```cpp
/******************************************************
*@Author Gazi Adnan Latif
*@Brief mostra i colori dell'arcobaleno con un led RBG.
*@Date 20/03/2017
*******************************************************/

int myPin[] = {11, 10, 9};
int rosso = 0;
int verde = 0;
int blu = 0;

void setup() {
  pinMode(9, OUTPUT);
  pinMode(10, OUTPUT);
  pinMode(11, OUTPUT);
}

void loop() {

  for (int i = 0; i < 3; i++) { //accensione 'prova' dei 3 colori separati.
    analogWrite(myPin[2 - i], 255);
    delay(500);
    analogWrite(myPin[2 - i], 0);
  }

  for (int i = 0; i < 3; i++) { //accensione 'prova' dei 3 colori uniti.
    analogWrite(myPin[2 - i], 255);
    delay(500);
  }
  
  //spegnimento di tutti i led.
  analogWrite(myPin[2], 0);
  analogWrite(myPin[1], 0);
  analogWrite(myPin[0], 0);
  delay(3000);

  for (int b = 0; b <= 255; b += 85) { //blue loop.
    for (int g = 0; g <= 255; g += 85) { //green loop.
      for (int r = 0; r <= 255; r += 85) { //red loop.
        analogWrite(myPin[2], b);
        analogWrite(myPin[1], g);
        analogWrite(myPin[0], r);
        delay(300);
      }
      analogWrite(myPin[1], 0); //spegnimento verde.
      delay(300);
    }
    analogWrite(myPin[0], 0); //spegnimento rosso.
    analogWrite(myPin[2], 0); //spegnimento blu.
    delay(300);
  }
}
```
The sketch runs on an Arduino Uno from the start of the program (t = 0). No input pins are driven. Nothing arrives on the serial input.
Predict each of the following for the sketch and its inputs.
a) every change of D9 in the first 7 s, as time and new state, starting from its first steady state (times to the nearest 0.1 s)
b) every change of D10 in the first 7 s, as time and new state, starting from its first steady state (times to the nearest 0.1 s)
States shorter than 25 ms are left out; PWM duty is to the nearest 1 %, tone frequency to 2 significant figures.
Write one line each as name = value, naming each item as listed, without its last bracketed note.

every change of D9 in the first 7 s, as time and new state, starting from its first steady state = 0 s high; 0.5 s low; 1.5 s high; 3 s low
every change of D10 in the first 7 s, as time and new state, starting from its first steady state = 0 s low; 0.5 s high; 1 s low; 2 s high; 3 s low
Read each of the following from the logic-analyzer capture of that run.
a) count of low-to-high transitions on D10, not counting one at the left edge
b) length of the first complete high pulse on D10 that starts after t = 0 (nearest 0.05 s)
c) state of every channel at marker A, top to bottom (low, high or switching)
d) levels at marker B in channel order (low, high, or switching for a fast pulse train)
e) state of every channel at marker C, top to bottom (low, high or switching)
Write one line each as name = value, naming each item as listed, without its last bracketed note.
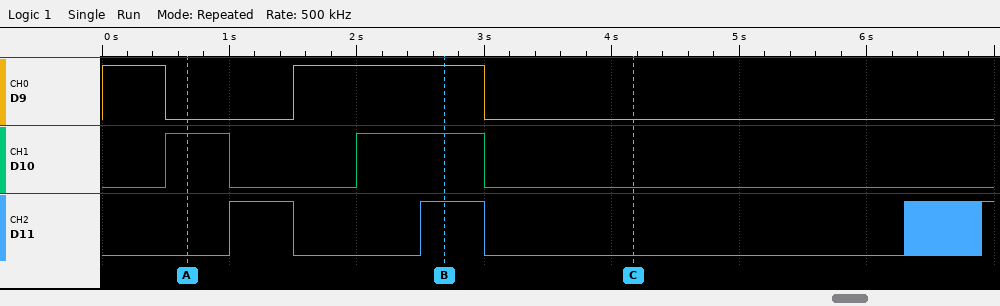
count of low-to-high transitions on D10, not counting one at the left edge = 2
length of the first complete high pulse on D10 that starts after t = 0 = 0.50 s
state of every channel at marker A, top to bottom = D9 low, D10 high, D11 low
levels at marker B in channel order = D9 high, D10 high, D11 high
state of every channel at marker C, top to bottom = D9 low, D10 low, D11 low
